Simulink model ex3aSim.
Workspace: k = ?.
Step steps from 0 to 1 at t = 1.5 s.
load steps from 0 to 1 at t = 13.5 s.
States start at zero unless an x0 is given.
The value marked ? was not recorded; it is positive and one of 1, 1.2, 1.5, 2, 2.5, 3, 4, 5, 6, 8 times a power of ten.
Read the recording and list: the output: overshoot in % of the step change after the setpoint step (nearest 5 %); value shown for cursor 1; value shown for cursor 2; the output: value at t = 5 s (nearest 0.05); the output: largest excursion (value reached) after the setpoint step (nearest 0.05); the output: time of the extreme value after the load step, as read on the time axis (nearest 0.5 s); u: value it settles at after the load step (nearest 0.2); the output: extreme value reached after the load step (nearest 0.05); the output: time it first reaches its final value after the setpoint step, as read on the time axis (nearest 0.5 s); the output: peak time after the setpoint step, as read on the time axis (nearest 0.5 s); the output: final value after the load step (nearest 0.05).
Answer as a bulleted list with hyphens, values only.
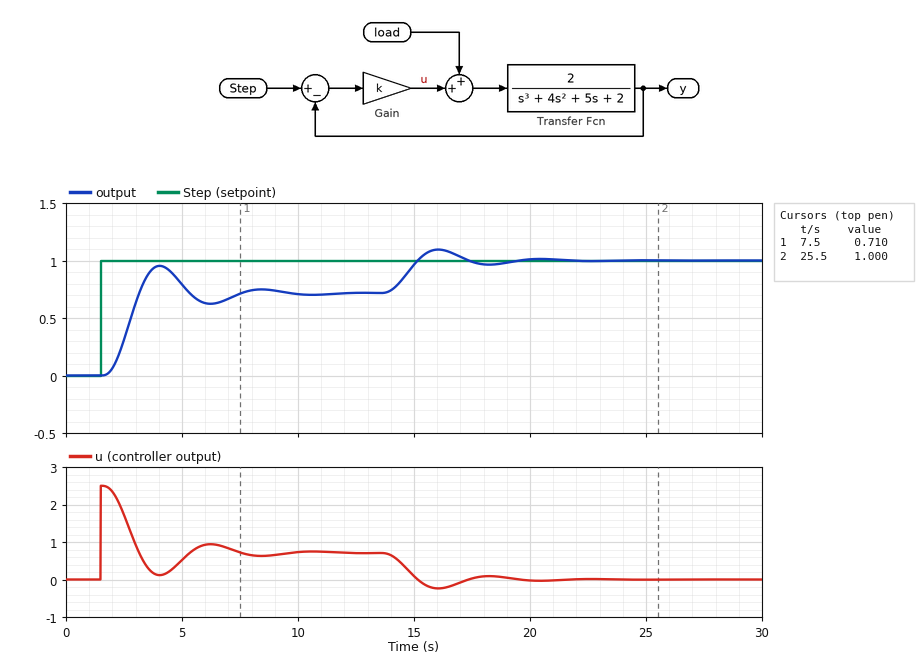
- 35 %
- 0.710
- 1.000
- 0.80
- 0.95
- 16.0 s
- 0.0
- 1.10
- 3.0 s
- 4.0 s
- 1.00
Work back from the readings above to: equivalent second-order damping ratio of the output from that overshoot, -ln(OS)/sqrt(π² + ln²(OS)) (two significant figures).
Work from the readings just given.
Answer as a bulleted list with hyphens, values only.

- 0.32
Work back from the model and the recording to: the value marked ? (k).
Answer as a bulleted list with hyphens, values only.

- 2.5
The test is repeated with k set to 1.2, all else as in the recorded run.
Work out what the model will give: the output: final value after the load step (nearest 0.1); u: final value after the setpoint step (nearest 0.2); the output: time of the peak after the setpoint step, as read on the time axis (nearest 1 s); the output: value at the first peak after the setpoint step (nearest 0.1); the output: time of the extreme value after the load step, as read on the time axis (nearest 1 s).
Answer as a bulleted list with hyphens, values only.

- 1.0
- 0.6
- 5 s
- 0.6
- 17 s
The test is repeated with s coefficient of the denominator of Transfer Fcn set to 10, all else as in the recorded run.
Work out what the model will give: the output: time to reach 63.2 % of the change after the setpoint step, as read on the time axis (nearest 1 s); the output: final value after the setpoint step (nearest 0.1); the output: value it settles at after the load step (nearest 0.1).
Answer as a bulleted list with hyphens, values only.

- 3 s
- 0.7
- 1.0
